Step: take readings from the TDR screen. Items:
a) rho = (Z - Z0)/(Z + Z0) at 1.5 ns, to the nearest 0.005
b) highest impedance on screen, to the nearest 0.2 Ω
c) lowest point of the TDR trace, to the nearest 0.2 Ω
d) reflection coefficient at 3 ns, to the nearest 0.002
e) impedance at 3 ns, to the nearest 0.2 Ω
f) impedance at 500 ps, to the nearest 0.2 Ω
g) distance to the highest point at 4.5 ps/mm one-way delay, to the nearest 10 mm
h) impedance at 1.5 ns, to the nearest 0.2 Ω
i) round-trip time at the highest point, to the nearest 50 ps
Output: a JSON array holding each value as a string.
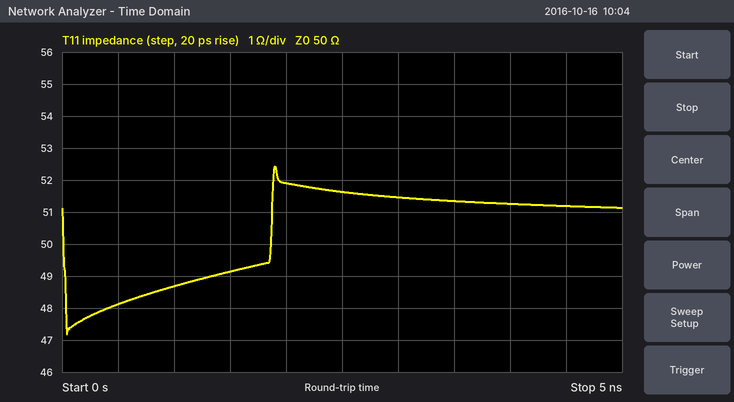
["-0.010", "52.4 Ω", "47.2 Ω", "+0.014", "51.4 Ω", "48.2 Ω", "210 mm", "49.2 Ω", "1.90 ns"]
